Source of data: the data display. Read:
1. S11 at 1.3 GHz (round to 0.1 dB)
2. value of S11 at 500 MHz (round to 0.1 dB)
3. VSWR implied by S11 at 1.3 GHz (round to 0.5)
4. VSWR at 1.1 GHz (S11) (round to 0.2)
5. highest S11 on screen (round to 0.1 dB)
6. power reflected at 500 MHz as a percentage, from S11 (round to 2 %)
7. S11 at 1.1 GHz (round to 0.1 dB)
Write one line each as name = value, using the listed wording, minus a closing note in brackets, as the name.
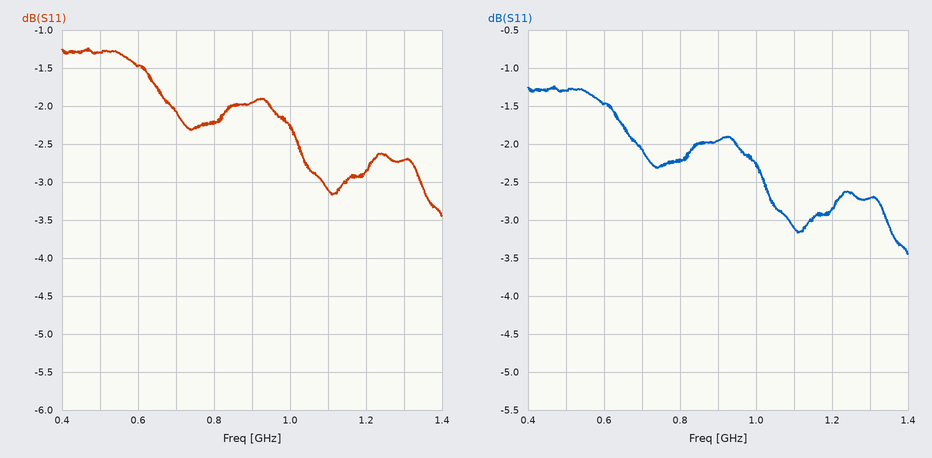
S11 at 1.3 GHz = -2.7 dB
value of S11 at 500 MHz = -1.3 dB
VSWR implied by S11 at 1.3 GHz = 6.5
VSWR at 1.1 GHz (S11) = 5.6
highest S11 on screen = -1.2 dB
power reflected at 500 MHz as a percentage, from S11 = 74 %
S11 at 1.1 GHz = -3.1 dB
